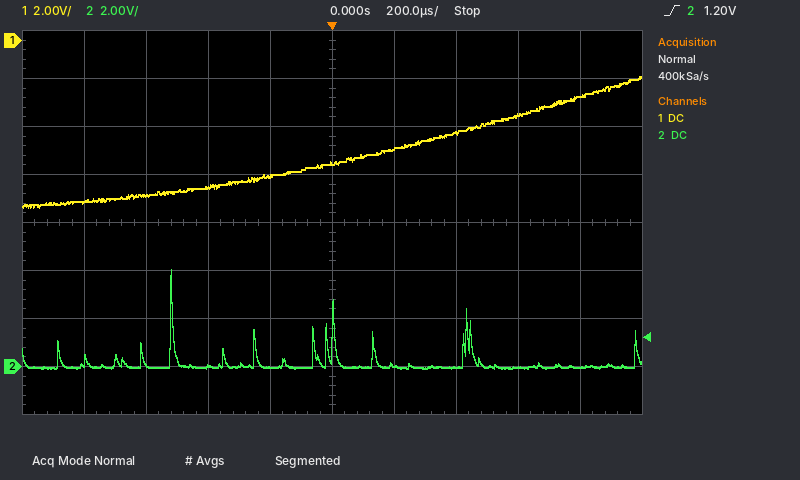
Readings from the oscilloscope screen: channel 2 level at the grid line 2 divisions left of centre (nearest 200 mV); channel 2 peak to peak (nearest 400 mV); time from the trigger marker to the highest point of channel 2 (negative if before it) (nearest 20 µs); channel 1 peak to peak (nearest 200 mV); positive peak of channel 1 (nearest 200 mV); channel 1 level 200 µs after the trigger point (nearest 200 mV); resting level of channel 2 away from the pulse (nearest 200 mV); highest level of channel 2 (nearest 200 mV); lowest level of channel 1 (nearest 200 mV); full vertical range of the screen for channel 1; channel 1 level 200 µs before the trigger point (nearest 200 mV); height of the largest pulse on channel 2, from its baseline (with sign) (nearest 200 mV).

0.0 V
4.0 V
-520 µs
5.4 V
-1.6 V
-4.6 V
0.0 V
4.0 V
-7.0 V
16 V
-5.6 V
+4.0 V
